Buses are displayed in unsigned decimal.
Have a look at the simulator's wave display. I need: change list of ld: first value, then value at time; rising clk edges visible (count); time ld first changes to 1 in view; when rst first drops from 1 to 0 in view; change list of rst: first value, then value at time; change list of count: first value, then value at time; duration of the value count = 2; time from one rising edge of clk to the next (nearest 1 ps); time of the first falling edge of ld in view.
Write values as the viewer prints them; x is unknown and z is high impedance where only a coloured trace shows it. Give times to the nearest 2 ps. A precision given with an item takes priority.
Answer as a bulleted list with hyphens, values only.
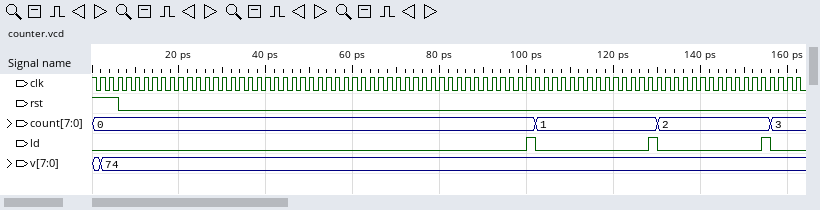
- 0, 1 at 100 ps, 0 at 102 ps, 1 at 128 ps, 0 at 130 ps, 1 at 154 ps, 0 at 156 ps
- 81
- 100 ps
- 6 ps
- 1, 0 at 6 ps
- 0, 1 at 102 ps, 2 at 130 ps, 3 at 156 ps
- 26 ps
- 2 ps
- 102 ps
